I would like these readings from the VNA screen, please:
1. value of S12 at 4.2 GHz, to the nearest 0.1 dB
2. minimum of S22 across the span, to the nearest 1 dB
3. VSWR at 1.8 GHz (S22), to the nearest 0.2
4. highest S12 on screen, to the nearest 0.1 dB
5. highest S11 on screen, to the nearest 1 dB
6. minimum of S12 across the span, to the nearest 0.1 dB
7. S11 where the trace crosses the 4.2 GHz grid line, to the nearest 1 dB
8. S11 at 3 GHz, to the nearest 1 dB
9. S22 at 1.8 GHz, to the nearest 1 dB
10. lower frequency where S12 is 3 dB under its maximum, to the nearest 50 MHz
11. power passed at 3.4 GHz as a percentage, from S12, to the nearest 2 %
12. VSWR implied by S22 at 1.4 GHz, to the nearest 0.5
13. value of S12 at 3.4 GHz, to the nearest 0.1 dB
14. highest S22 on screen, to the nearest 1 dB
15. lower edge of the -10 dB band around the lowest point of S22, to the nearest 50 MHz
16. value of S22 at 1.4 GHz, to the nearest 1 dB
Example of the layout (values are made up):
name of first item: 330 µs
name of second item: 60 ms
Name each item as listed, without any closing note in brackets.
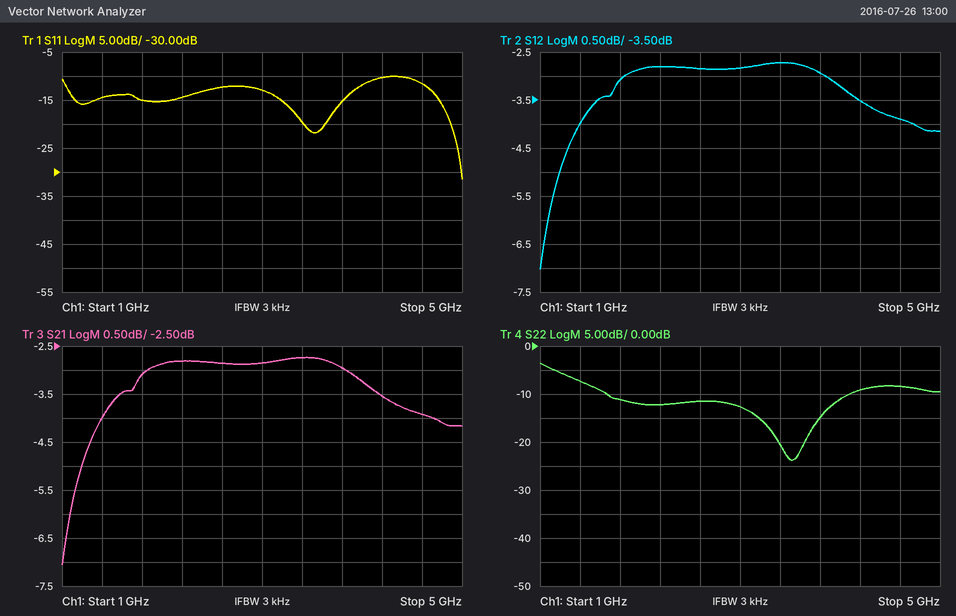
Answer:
value of S12 at 4.2 GHz, to the nearest 0.1 dB: -3.5 dB
minimum of S22 across the span, to the nearest 1 dB: -24 dB
VSWR at 1.8 GHz (S22), to the nearest 0.2: 1.8
highest S12 on screen, to the nearest 0.1 dB: -2.7 dB
highest S11 on screen, to the nearest 1 dB: -10 dB
minimum of S12 across the span, to the nearest 0.1 dB: -7.0 dB
S11 where the trace crosses the 4.2 GHz grid line, to the nearest 1 dB: -10 dB
S11 at 3 GHz, to the nearest 1 dB: -13 dB
S22 at 1.8 GHz, to the nearest 1 dB: -11 dB
lower frequency where S12 is 3 dB under its maximum, to the nearest 50 MHz: 1.10 GHz
power passed at 3.4 GHz as a percentage, from S12, to the nearest 2 %: 54 %
VSWR implied by S22 at 1.4 GHz, to the nearest 0.5: 2.5
value of S12 at 3.4 GHz, to the nearest 0.1 dB: -2.7 dB
highest S22 on screen, to the nearest 1 dB: -4 dB
lower edge of the -10 dB band around the lowest point of S22, to the nearest 50 MHz: 1.65 GHz
value of S22 at 1.4 GHz, to the nearest 1 dB: -7 dB
